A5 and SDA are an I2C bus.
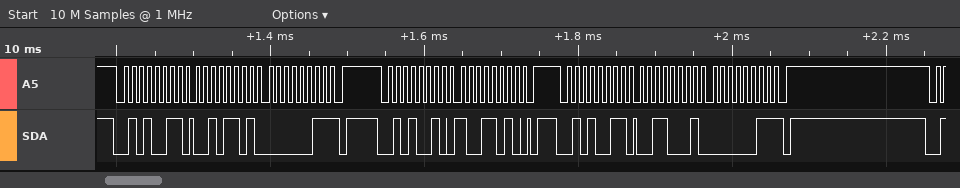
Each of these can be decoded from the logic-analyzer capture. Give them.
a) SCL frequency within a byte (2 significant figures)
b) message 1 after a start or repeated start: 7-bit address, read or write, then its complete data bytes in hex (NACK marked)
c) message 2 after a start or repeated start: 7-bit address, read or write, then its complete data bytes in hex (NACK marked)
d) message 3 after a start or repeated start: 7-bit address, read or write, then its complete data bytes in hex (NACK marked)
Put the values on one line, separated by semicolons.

100 kHz; 0x29 read: 2D 03 NACK; 0x29 write: 9A; 0x29 read: 31 03 NACK
